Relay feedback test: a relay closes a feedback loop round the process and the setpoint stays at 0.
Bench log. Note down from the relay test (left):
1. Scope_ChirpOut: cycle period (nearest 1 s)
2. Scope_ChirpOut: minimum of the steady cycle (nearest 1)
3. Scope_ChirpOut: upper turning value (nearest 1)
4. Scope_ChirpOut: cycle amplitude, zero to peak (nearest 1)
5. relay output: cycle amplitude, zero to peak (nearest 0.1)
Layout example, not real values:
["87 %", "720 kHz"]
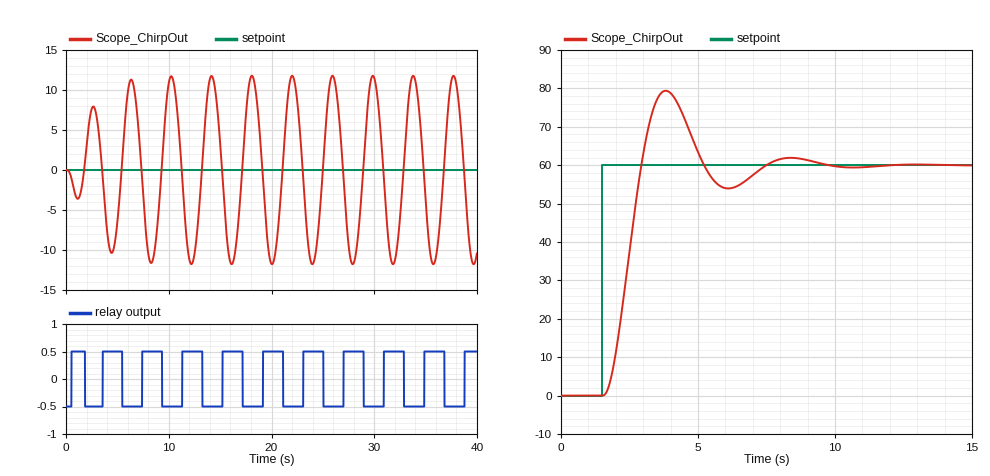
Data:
["4 s", "-12", "12", "12", "0.5"]
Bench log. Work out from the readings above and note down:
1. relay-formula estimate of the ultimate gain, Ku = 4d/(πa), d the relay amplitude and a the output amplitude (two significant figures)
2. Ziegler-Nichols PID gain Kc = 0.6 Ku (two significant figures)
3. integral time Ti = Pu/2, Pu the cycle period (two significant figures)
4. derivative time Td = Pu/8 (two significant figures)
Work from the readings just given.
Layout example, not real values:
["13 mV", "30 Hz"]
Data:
["0.053", "0.032", "2.0 s", "0.50 s"]
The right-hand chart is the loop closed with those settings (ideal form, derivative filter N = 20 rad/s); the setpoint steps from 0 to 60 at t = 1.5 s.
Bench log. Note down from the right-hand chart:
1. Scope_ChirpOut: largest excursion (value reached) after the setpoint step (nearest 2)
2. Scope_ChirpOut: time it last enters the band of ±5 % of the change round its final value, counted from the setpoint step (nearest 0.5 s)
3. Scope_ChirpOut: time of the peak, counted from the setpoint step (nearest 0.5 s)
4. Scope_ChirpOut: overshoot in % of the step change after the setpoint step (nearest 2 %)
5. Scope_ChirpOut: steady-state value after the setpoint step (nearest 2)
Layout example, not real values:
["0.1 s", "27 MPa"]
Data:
["80", "5.5 s", "2.5 s", "32 %", "60"]
